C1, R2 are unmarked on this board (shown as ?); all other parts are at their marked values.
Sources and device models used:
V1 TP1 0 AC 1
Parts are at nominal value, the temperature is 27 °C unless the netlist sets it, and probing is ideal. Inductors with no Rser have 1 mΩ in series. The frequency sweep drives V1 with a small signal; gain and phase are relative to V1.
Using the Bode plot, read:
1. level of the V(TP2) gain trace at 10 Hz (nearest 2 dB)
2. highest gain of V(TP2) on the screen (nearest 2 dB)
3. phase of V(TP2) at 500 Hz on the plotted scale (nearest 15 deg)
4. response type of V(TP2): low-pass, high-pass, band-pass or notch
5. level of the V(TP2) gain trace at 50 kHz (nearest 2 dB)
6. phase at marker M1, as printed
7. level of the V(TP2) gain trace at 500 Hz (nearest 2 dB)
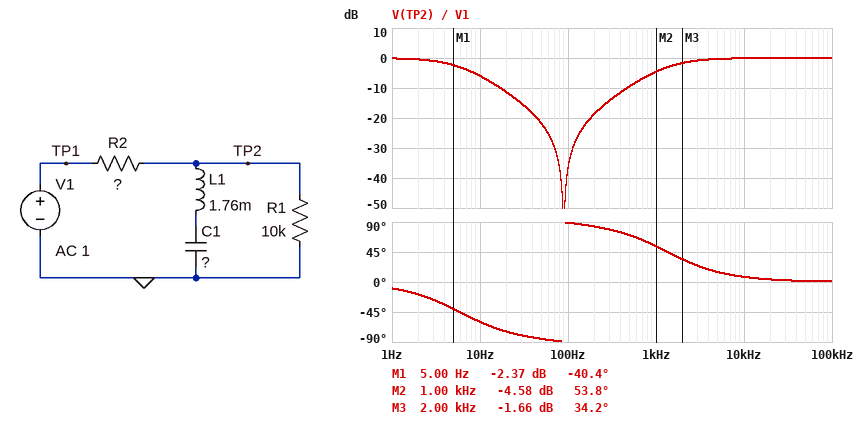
-6 dB
0 dB
75 deg
notch
0 dB
-40.4 deg
-10 dB
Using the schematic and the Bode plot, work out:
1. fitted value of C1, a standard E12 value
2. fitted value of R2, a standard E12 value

1.8 mF
15 Ω
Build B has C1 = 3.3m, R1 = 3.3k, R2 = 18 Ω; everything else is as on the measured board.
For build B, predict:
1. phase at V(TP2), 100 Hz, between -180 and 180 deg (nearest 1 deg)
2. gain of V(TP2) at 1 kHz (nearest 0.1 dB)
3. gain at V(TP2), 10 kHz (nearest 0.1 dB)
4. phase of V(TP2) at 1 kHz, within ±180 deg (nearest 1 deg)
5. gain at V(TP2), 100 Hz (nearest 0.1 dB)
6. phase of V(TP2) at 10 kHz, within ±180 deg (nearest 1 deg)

88 deg
-5.7 dB
-0.2 dB
58 deg
-29.2 dB
9 deg
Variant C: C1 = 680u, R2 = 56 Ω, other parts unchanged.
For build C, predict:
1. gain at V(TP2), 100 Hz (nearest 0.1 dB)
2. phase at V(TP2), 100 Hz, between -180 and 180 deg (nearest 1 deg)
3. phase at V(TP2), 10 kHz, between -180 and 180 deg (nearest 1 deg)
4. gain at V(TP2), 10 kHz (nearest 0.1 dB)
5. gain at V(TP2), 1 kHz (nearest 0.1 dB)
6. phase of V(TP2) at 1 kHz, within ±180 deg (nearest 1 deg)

-33.1 dB
-89 deg
27 deg
-1.0 dB
-14.4 dB
79 deg
